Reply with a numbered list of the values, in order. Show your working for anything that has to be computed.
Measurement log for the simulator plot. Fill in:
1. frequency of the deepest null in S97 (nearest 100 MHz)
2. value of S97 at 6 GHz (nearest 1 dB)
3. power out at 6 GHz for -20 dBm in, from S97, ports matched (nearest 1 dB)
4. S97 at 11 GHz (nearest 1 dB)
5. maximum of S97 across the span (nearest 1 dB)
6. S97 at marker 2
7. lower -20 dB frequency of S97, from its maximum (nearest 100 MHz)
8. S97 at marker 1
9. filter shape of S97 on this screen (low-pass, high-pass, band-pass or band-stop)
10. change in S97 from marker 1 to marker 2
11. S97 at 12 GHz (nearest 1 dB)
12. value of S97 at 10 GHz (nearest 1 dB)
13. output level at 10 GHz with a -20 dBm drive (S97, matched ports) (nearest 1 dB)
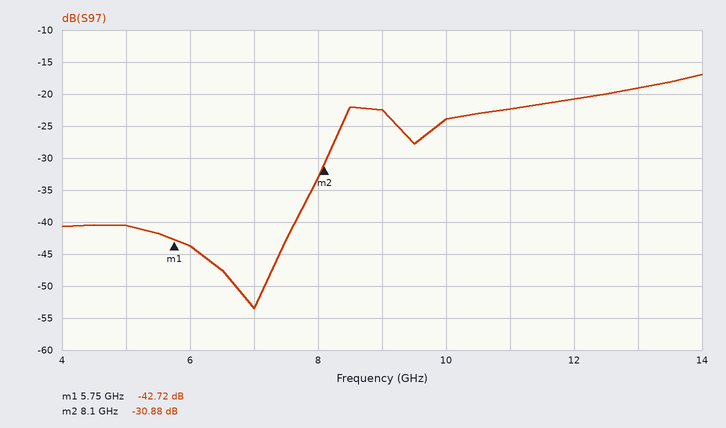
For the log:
1. 7.0 GHz
2. -44 dB
3. -20 dBm + (-44 dB) = -64 dBm
4. -22 dB
5. -17 dB
6. -30.88 dB
7. 7.8 GHz
8. -42.72 dB
9. high-pass
10. -30.88 − (-42.72) = 11.84 dB
11. -21 dB
12. -24 dB
13. -20 dBm + (-24 dB) = -44 dBm
